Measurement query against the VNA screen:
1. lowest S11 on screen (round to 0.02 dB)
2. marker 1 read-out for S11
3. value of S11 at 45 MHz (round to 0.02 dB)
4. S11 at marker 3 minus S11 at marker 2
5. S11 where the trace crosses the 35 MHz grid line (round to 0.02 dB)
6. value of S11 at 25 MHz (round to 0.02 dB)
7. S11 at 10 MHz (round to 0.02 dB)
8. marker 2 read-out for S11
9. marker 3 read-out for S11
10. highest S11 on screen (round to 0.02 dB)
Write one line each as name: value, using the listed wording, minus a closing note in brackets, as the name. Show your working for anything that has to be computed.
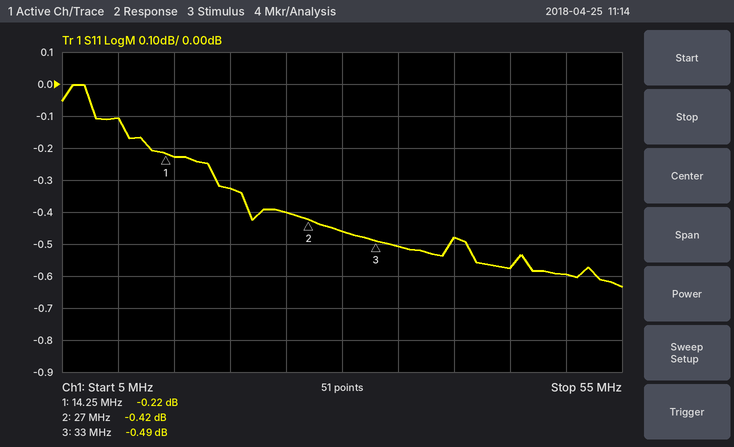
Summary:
lowest S11 on screen: -0.64 dB
marker 1 read-out for S11: -0.22 dB
value of S11 at 45 MHz: -0.58 dB
S11 at marker 3 minus S11 at marker 2: -0.49 − (-0.42) = -0.07 dB
S11 where the trace crosses the 35 MHz grid line: -0.50 dB
value of S11 at 25 MHz: -0.40 dB
S11 at 10 MHz: -0.10 dB
marker 2 read-out for S11: -0.42 dB
marker 3 read-out for S11: -0.49 dB
highest S11 on screen: 0.00 dB
